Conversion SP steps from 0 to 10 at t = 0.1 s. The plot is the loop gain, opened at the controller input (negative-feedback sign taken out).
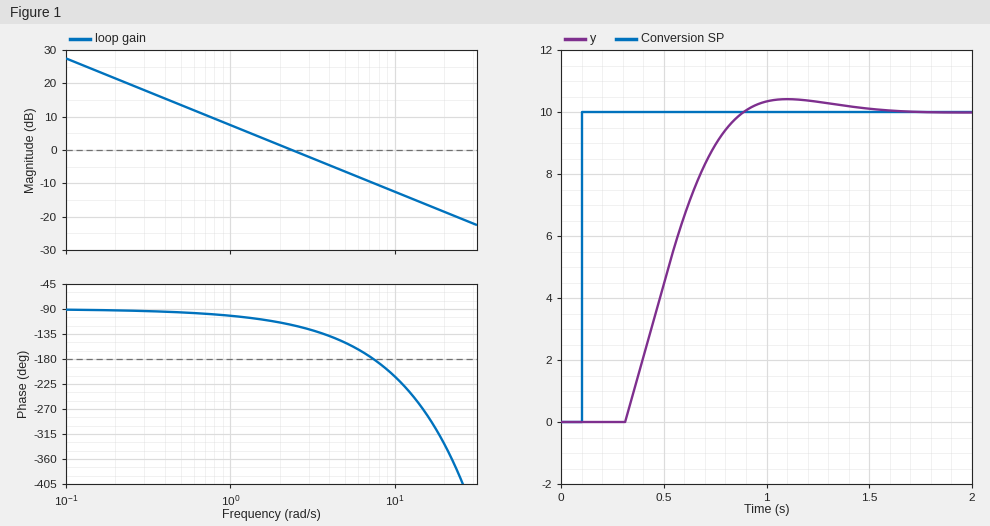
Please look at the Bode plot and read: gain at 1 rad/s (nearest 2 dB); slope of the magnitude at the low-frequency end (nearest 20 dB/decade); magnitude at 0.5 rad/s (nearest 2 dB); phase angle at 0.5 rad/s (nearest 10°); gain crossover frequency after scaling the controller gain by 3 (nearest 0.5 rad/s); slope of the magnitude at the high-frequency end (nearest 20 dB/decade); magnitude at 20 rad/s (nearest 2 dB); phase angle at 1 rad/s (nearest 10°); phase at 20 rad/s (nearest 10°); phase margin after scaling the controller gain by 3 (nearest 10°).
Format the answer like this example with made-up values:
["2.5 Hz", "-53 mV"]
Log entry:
["8 dB", "-20 dB/decade", "14 dB", "-100°", "7.0 rad/s", "-20 dB/decade", "-18 dB", "-100°", "-330°", "0°"]
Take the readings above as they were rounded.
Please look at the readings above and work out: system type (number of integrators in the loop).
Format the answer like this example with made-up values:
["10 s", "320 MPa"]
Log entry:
["1"]
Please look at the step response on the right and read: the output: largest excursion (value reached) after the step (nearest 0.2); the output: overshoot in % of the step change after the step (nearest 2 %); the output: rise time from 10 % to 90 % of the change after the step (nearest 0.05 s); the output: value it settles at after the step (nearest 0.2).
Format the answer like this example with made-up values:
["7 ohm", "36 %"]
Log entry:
["10.4", "4 %", "0.40 s", "10.0"]
